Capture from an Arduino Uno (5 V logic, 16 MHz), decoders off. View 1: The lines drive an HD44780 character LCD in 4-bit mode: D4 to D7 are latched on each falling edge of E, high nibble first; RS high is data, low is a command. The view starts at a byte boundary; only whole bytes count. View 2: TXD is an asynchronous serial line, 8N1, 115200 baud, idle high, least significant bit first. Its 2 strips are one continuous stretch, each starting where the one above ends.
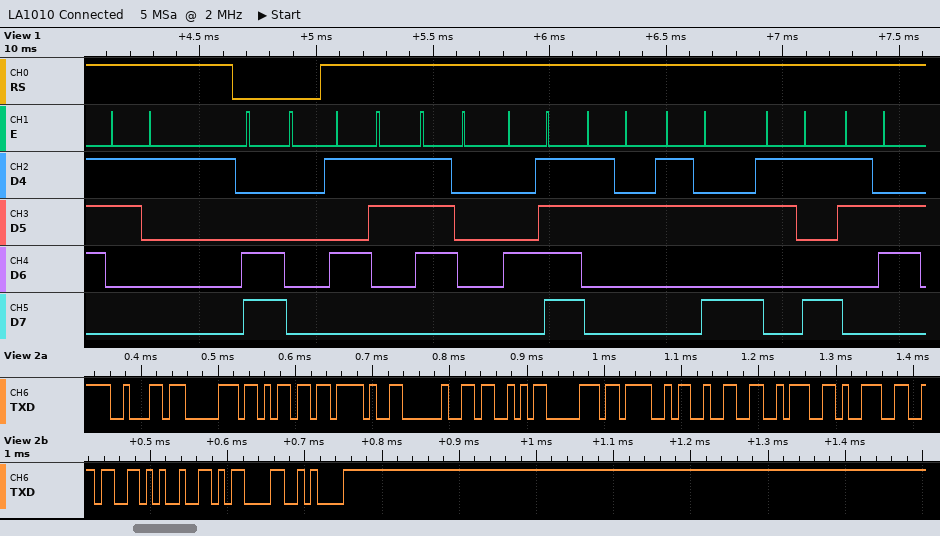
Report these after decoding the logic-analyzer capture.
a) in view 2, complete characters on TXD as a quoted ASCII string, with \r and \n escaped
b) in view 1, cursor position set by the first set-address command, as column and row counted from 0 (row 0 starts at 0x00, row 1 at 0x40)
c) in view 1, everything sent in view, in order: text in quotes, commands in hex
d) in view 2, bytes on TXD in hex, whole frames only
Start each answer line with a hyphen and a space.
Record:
- "bpm/ SpO2:96%\r\n"
- column 0, row 1
- "1" 0xC0 "SpO2:96"
- 62 70 6D 2F 20 53 70 4F 32 3A 39 36 25 0D 0A
